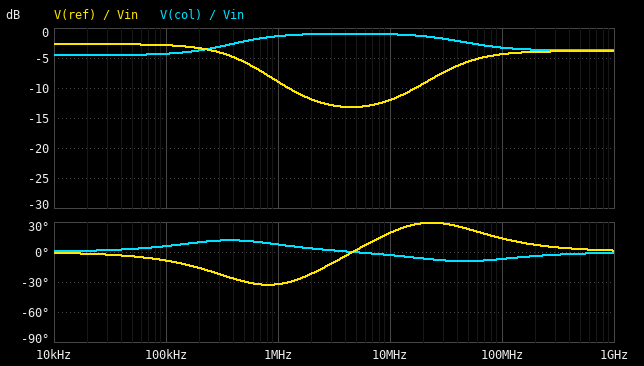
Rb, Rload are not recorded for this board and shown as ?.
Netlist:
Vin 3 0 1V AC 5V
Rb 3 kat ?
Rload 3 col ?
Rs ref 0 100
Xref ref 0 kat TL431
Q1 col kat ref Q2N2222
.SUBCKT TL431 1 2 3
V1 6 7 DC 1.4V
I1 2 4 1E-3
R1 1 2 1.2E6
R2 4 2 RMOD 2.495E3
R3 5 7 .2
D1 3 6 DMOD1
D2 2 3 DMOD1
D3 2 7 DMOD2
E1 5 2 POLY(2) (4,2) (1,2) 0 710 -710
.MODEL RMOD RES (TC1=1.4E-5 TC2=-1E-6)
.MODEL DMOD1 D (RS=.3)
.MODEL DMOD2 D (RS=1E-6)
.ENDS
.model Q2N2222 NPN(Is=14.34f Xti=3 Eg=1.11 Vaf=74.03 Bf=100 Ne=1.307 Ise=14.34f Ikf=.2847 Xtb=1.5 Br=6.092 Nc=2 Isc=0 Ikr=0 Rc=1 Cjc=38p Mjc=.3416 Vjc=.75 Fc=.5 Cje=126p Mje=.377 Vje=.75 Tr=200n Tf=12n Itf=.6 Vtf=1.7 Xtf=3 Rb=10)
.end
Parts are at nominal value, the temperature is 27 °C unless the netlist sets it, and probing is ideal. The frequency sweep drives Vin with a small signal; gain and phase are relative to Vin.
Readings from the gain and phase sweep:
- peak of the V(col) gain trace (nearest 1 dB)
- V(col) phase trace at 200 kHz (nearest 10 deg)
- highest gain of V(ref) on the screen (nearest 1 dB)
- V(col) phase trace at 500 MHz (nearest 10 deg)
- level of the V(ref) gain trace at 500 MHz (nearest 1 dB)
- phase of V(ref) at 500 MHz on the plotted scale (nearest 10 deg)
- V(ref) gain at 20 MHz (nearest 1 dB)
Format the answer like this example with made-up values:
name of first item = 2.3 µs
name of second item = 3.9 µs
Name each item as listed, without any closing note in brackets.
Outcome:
peak of the V(col) gain trace = -1 dB
V(col) phase trace at 200 kHz = 10 deg
highest gain of V(ref) on the screen = -3 dB
V(col) phase trace at 500 MHz = 0 deg
level of the V(ref) gain trace at 500 MHz = -4 dB
phase of V(ref) at 500 MHz on the plotted scale = 0 deg
V(ref) gain at 20 MHz = -9 dB
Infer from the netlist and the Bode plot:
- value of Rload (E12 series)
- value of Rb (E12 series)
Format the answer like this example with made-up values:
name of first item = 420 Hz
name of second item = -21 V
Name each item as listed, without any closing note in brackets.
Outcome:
value of Rload = 56 Ω
value of Rb = 2.2 kΩ
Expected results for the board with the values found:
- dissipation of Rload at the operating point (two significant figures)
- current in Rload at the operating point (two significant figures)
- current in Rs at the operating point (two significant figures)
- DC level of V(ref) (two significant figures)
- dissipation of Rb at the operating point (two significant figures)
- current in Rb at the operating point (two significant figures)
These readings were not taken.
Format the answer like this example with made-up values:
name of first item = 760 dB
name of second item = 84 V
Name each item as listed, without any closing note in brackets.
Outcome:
dissipation of Rload at the operating point = 370 µW
current in Rload at the operating point = 2.6 mA
current in Rs at the operating point = 2.6 mA
DC level of V(ref) = 260 mV
dissipation of Rb at the operating point = 2.2 µW
current in Rb at the operating point = 32 µA
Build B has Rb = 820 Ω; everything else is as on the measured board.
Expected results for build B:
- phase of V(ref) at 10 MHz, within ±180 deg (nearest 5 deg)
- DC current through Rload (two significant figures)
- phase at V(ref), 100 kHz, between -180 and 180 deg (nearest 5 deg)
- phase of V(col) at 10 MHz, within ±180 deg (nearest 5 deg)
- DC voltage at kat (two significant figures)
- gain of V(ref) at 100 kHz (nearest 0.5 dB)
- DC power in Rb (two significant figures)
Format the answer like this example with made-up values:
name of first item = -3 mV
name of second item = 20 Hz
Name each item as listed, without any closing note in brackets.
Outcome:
phase of V(ref) at 10 MHz, within ±180 deg = 10 deg
DC current through Rload = 2.9 mA
phase at V(ref), 100 kHz, between -180 and 180 deg = -5 deg
phase of V(col) at 10 MHz, within ±180 deg = 0 deg
DC voltage at kat = 970 mV
gain of V(ref) at 100 kHz = -1.5 dB
DC power in Rb = 1.1 µW
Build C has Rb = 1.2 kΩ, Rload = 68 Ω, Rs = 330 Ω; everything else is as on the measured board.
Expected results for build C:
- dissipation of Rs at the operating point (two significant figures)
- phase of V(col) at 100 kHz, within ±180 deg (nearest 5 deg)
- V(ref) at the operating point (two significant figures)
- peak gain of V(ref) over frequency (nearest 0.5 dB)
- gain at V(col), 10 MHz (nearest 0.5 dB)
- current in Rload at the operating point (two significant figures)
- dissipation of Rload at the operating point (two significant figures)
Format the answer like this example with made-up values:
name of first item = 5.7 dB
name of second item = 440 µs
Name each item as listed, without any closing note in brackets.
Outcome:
dissipation of Rs at the operating point = 350 µW
phase of V(col) at 100 kHz, within ±180 deg = 0 deg
V(ref) at the operating point = 340 mV
peak gain of V(ref) over frequency = -1.0 dB
gain at V(col), 10 MHz = -0.5 dB
current in Rload at the operating point = 1.0 mA
dissipation of Rload at the operating point = 70 µW
